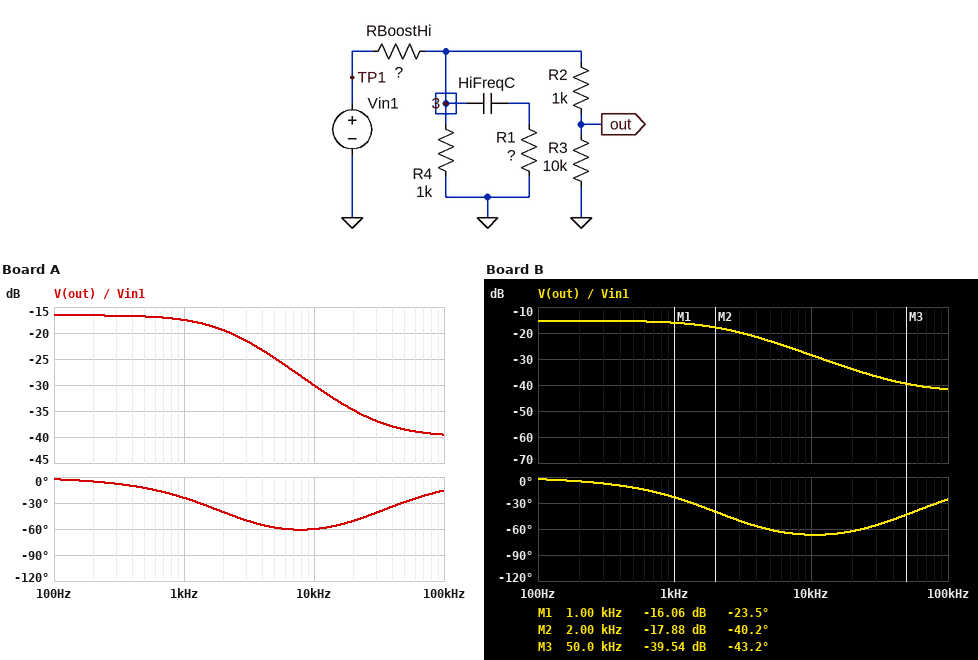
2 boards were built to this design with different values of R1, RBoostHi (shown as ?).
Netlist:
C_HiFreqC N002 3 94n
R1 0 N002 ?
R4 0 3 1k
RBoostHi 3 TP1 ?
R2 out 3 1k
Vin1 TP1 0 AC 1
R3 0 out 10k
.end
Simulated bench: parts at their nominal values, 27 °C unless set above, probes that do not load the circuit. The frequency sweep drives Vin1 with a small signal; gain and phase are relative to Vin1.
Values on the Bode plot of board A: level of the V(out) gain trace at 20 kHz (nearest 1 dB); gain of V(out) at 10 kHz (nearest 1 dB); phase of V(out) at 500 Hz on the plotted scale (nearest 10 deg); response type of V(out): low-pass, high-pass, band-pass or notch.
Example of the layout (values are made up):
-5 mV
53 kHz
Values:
-35 dB
-30 dB
-10 deg
low-pass
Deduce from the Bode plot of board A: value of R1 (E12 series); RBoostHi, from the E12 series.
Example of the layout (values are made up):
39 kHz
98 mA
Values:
56 Ω
4.7 kΩ
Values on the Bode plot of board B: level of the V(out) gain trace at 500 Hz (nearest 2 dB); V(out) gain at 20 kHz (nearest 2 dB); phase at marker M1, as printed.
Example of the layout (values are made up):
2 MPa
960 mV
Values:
-16 dB
-34 dB
-23.5 deg
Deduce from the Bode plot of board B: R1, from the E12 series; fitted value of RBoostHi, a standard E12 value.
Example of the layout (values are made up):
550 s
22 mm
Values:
33 Ω
3.9 kΩ
